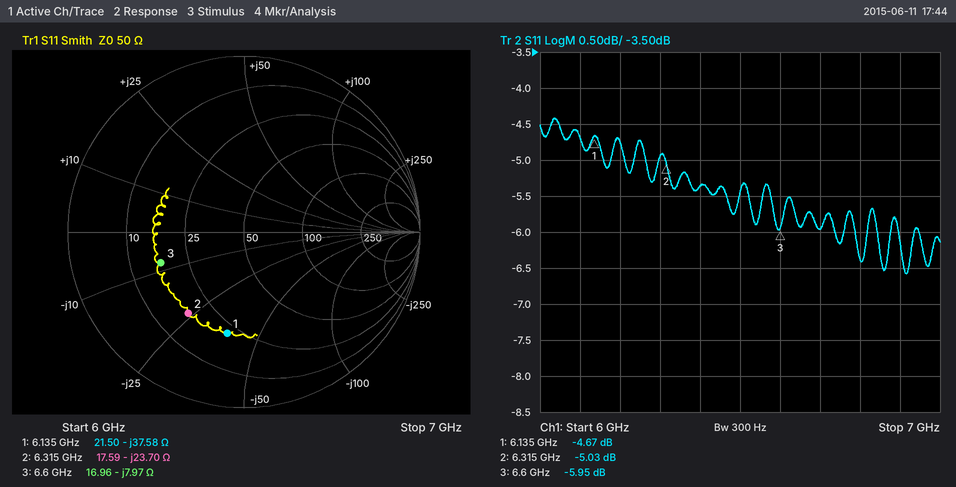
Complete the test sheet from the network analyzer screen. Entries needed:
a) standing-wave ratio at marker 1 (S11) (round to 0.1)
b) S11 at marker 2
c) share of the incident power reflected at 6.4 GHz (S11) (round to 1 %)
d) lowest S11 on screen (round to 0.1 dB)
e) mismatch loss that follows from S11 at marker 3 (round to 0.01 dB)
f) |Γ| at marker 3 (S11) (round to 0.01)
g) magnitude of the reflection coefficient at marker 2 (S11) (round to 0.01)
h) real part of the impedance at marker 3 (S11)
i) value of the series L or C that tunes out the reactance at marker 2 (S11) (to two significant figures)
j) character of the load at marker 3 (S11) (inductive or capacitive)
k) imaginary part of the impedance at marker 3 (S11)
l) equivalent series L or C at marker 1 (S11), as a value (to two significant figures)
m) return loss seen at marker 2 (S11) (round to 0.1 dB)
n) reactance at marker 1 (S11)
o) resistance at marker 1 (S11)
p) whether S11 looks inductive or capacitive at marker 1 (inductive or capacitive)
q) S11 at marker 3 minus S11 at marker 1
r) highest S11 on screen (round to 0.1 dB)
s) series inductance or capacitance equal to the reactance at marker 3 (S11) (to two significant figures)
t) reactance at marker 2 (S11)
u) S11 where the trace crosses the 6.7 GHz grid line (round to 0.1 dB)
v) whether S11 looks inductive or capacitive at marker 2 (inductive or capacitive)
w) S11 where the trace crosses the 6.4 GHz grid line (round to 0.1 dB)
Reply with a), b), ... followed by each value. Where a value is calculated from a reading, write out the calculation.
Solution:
a) 3.8
b) -5.03 dB
c) 10^(-5.4/10) ≈ 29 %
d) -6.6 dB
e) −10 log10(1 − 10^(-5.95/10)) ≈ 1.27 dB
f) 0.50
g) 10^(-5.03/20) ≈ 0.56
h) 16.96 Ω
i) L = 23.7 Ω/(2π × 6.315 GHz) ≈ 597 pH, so 600 pH to two significant figures
j) capacitive
k) -7.97 Ω
l) C = 1/(2π × 6.135 GHz × 37.58 Ω) ≈ 690 fF
m) 5.0 dB
n) -37.58 Ω
o) 21.50 Ω
p) capacitive
q) -5.95 − (-4.67) = -1.28 dB
r) -4.4 dB
s) C = 1/(2π × 6.6 GHz × 7.97 Ω) ≈ 3.0 pF
t) -23.70 Ω
u) -6.0 dB
v) capacitive
w) -5.4 dB
